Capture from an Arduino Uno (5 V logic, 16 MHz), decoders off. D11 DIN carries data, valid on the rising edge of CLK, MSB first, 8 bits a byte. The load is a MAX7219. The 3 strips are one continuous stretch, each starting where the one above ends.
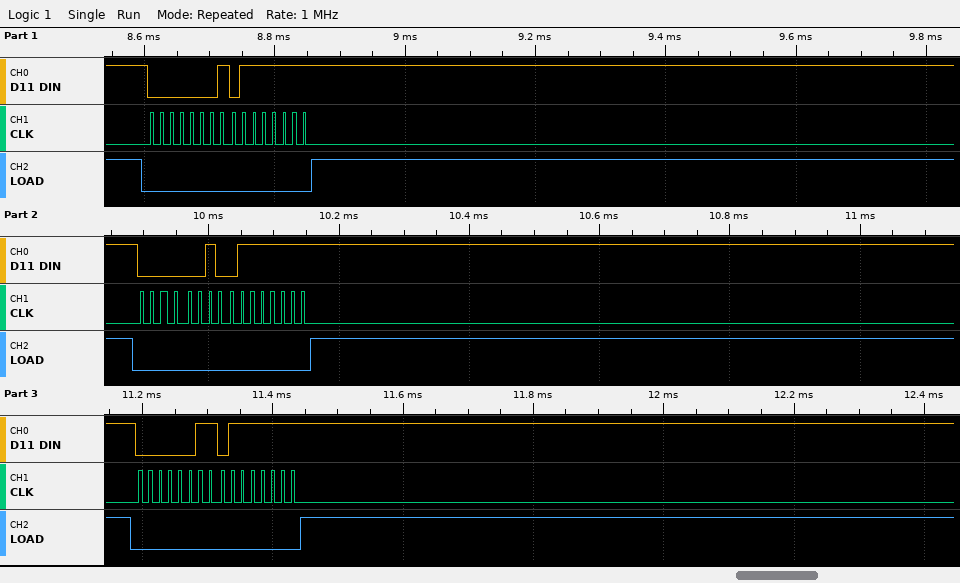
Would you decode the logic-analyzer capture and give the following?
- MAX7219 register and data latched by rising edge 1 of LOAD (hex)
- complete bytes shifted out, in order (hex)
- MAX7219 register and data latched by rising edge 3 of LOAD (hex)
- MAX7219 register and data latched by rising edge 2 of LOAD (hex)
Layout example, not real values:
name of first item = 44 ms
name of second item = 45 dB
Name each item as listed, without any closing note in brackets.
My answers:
MAX7219 register and data latched by rising edge 1 of LOAD = register 0x1, data 0x7F
complete bytes shifted out, in order = 01 7F 02 7F 03 7F
MAX7219 register and data latched by rising edge 3 of LOAD = register 0x3, data 0x7F
MAX7219 register and data latched by rising edge 2 of LOAD = register 0x2, data 0x7F
